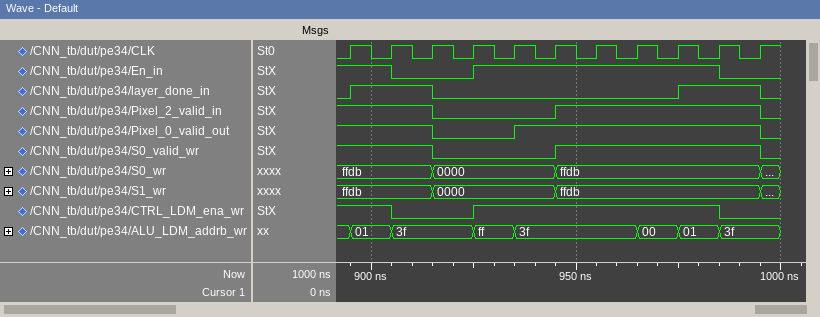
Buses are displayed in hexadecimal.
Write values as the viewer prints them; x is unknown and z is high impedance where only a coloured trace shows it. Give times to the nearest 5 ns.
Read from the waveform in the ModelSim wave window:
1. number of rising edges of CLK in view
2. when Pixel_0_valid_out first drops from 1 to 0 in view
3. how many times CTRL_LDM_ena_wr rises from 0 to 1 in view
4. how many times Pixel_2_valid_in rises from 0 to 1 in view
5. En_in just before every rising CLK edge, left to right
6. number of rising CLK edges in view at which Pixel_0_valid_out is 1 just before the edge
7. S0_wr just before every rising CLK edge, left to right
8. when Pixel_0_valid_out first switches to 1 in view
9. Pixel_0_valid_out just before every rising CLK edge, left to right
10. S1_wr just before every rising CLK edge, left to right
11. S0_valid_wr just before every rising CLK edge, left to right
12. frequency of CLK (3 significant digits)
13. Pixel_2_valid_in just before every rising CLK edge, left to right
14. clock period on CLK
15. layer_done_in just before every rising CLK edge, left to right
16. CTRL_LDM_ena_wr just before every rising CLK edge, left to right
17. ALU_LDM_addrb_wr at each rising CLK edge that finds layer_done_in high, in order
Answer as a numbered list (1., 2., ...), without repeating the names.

1. 11
2. 915 ns
3. 1
4. 1
5. 1 1 0 0 1 1 1 1 1 1 0
6. 9
7. ffdb, ffdb, ffdb, 0000, 0000, 0000, ffdb, ffdb, ffdb, ffdb, ffdb
8. 935 ns
9. 1 1 1 0 0 1 1 1 1 1 1
10. ffdb, ffdb, ffdb, 0000, 0000, 0000, ffdb, ffdb, ffdb, ffdb, ffdb
11. 1 1 1 0 0 0 1 1 1 1 1
12. 100 MHz
13. 1 1 1 0 0 0 1 1 1 1 1
14. 10 ns
15. 0 1 1 0 0 0 0 0 0 1 1
16. 1 1 0 0 1 1 1 1 1 1 0
17. 01, 3f, 01, 3f
